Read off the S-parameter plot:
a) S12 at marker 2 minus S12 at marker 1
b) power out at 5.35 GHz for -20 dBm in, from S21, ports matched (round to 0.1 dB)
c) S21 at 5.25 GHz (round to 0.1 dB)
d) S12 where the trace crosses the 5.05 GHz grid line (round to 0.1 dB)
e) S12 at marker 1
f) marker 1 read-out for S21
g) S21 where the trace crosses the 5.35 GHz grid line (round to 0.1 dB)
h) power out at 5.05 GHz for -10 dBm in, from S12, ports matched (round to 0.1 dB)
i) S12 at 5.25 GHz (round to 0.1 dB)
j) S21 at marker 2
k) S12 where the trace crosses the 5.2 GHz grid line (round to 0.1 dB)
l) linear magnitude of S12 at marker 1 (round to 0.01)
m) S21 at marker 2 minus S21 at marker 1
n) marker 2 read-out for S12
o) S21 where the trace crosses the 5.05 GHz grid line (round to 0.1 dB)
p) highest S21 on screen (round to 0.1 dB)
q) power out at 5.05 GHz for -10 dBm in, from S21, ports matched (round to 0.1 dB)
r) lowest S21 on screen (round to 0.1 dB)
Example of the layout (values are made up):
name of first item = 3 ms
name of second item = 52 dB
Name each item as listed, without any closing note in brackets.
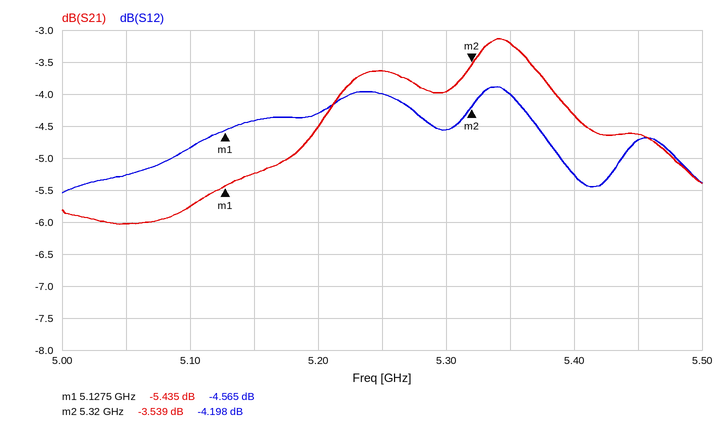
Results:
S12 at marker 2 minus S12 at marker 1 = 0.367 dB
power out at 5.35 GHz for -20 dBm in, from S21, ports matched = -23.2 dBm
S21 at 5.25 GHz = -3.6 dB
S12 where the trace crosses the 5.05 GHz grid line = -5.3 dB
S12 at marker 1 = -4.565 dB
marker 1 read-out for S21 = -5.435 dB
S21 where the trace crosses the 5.35 GHz grid line = -3.2 dB
power out at 5.05 GHz for -10 dBm in, from S12, ports matched = -15.3 dBm
S12 at 5.25 GHz = -4.0 dB
S21 at marker 2 = -3.539 dB
S12 where the trace crosses the 5.2 GHz grid line = -4.3 dB
linear magnitude of S12 at marker 1 = 0.59
S21 at marker 2 minus S21 at marker 1 = 1.896 dB
marker 2 read-out for S12 = -4.198 dB
S21 where the trace crosses the 5.05 GHz grid line = -6.0 dB
highest S21 on screen = -3.1 dB
power out at 5.05 GHz for -10 dBm in, from S21, ports matched = -16.0 dBm
lowest S21 on screen = -6.0 dB
